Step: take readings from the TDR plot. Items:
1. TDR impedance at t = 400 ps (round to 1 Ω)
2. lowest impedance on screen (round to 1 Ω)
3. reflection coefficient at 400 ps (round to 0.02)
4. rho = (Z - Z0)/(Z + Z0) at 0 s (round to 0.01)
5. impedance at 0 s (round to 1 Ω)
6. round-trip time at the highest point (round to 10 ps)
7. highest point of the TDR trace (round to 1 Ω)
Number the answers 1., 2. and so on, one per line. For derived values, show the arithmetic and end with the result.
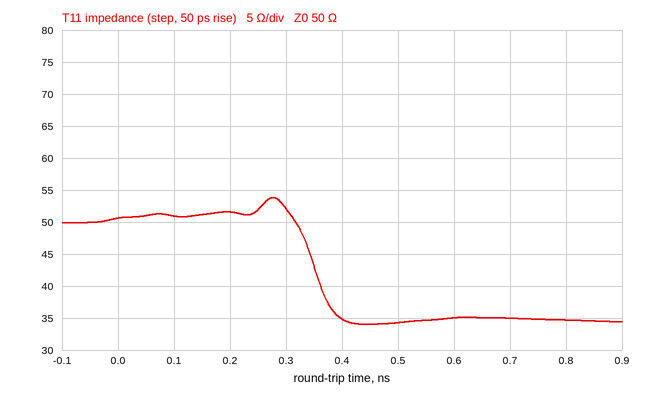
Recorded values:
1. 35 Ω
2. 34 Ω
3. (35 − 50)/(35 + 50) ≈ -0.18
4. (51 − 50)/(51 + 50) ≈ +0.01
5. 51 Ω
6. 280 ps
7. 54 Ω
